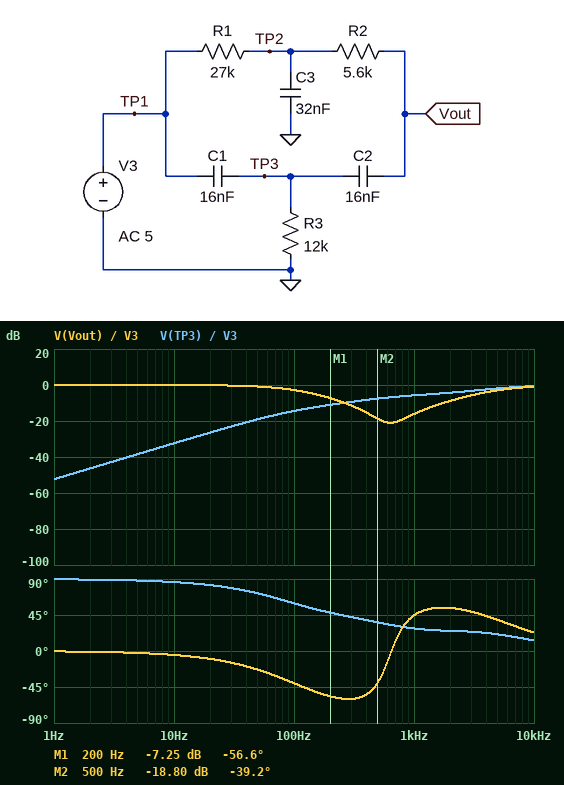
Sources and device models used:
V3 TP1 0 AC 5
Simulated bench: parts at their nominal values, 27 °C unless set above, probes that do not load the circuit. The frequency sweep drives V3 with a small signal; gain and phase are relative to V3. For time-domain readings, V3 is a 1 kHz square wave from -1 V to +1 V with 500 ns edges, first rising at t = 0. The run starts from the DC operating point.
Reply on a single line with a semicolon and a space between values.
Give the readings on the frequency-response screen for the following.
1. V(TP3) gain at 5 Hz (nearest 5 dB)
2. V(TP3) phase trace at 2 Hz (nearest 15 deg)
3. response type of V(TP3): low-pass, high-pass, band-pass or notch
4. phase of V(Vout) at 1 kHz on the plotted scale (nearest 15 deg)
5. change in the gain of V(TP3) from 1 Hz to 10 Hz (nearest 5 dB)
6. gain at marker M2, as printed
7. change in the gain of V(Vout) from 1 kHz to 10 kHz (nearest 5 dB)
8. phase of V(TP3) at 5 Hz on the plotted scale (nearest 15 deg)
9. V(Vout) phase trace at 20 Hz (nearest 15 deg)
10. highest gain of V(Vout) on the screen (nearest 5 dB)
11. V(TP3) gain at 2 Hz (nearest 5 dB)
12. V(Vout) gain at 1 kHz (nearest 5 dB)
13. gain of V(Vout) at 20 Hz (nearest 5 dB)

-40 dB; 90 deg; high-pass; 45 deg; 20 dB; -18.80 dB; 15 dB; 90 deg; -15 deg; 0 dB; -45 dB; -15 dB; 0 dB
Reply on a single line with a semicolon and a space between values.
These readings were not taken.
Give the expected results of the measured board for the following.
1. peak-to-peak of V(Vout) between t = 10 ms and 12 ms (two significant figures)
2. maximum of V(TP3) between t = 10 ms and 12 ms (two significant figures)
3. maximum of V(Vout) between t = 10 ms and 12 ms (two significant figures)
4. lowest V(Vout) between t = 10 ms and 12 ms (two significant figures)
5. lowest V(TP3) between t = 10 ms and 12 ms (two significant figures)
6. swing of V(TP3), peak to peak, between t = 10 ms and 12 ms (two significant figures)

3.6 V; 1.7 V; 1.8 V; -1.8 V; -1.7 V; 3.5 V
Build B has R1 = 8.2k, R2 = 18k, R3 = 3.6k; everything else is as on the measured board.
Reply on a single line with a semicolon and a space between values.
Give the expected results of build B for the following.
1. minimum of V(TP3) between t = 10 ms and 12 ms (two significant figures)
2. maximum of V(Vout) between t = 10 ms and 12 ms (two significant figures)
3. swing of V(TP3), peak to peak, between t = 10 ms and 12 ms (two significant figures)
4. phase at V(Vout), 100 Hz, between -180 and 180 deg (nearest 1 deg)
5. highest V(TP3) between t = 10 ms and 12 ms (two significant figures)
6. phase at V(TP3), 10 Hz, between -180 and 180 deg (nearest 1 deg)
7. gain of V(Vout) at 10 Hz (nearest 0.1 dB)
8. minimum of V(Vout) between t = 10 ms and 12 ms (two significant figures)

-1.9 V; 1.7 V; 3.8 V; -24 deg; 1.9 V; 88 deg; 0 dB; -1.7 V
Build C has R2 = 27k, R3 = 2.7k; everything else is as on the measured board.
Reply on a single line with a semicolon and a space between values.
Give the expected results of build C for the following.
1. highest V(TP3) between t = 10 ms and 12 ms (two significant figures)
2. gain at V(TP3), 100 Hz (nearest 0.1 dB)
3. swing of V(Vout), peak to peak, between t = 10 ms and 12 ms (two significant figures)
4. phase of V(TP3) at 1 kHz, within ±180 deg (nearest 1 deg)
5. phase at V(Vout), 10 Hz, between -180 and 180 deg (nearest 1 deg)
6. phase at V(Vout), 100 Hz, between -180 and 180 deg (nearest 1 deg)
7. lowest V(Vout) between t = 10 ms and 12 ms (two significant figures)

2.0 V; -27.6 dB; 3.9 V; 72 deg; -6 deg; -52 deg; -2.0 V
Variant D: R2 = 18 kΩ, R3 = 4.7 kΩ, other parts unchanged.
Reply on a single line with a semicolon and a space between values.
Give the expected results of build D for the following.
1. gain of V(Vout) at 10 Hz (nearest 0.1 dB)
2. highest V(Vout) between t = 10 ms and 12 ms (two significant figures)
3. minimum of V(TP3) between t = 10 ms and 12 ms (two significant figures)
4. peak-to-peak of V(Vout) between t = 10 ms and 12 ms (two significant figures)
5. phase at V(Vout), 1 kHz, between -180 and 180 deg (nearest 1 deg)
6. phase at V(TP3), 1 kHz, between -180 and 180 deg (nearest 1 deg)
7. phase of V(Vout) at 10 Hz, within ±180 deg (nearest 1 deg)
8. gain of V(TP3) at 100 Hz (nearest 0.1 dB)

0 dB; 1.9 V; -1.9 V; 3.9 V; 94 deg; 59 deg; -6 deg; -22.6 dB
